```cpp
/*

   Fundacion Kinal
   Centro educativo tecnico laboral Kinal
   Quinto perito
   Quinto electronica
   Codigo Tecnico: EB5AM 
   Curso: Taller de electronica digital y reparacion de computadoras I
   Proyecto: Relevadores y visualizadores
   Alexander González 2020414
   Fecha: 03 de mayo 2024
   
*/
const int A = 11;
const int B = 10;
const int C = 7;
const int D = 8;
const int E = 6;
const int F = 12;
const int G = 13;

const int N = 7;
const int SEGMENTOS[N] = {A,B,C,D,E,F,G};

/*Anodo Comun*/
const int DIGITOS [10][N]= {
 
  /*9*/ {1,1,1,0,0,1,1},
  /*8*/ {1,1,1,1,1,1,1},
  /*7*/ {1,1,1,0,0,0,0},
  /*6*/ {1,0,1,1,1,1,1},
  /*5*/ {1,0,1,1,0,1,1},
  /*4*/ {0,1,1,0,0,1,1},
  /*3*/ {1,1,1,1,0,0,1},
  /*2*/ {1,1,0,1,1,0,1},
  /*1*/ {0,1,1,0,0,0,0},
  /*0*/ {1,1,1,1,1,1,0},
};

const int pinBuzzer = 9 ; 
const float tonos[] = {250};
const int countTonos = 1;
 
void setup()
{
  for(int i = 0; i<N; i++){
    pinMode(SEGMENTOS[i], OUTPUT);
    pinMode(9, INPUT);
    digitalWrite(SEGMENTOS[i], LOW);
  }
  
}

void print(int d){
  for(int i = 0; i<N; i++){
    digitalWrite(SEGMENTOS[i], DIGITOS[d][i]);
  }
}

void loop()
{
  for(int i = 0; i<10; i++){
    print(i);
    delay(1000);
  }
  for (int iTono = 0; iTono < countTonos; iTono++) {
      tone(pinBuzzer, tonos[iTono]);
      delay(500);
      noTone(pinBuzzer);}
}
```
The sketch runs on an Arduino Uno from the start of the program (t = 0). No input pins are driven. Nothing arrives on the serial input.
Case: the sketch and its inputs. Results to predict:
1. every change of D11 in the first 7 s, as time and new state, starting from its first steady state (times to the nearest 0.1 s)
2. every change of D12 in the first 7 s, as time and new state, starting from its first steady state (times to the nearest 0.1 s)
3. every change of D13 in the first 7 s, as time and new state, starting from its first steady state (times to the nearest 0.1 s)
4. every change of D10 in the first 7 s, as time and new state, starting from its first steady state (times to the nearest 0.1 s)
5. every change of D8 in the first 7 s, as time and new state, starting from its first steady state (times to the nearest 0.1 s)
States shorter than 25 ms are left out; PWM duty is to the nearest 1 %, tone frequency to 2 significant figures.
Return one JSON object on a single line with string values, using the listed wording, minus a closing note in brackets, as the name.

{"every change of D11 in the first 7 s, as time and new state, starting from its first steady state": "0 s high; 5 s low; 6 s high", "every change of D12 in the first 7 s, as time and new state, starting from its first steady state": "0 s high; 2 s low; 3 s high; 6 s low", "every change of D13 in the first 7 s, as time and new state, starting from its first steady state": "0 s high; 2 s low; 3 s high", "every change of D10 in the first 7 s, as time and new state, starting from its first steady state": "0 s high; 3 s low; 5 s high", "every change of D8 in the first 7 s, as time and new state, starting from its first steady state": "0 s low; 1 s high; 2 s low; 3 s high; 5 s low; 6 s high"}
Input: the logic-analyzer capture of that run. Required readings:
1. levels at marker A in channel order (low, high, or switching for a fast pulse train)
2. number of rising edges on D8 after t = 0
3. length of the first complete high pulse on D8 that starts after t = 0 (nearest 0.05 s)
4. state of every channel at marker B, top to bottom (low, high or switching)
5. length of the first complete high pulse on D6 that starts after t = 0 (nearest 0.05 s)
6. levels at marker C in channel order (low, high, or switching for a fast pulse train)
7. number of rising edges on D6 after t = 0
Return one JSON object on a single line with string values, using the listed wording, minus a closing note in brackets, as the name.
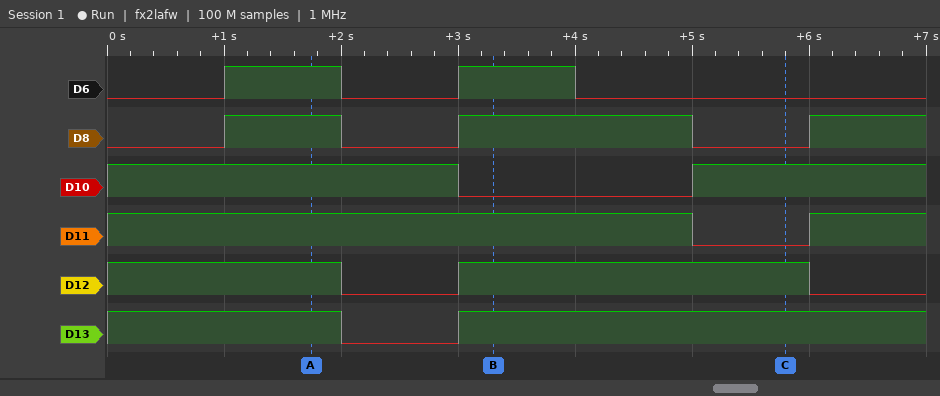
{"levels at marker A in channel order": "D6 high, D8 high, D10 high, D11 high, D12 high, D13 high", "number of rising edges on D8 after t = 0": "3", "length of the first complete high pulse on D8 that starts after t = 0": "1.00 s", "state of every channel at marker B, top to bottom": "D6 high, D8 high, D10 low, D11 high, D12 high, D13 high", "length of the first complete high pulse on D6 that starts after t = 0": "1.00 s", "levels at marker C in channel order": "D6 low, D8 low, D10 high, D11 low, D12 high, D13 high", "number of rising edges on D6 after t = 0": "2"}
